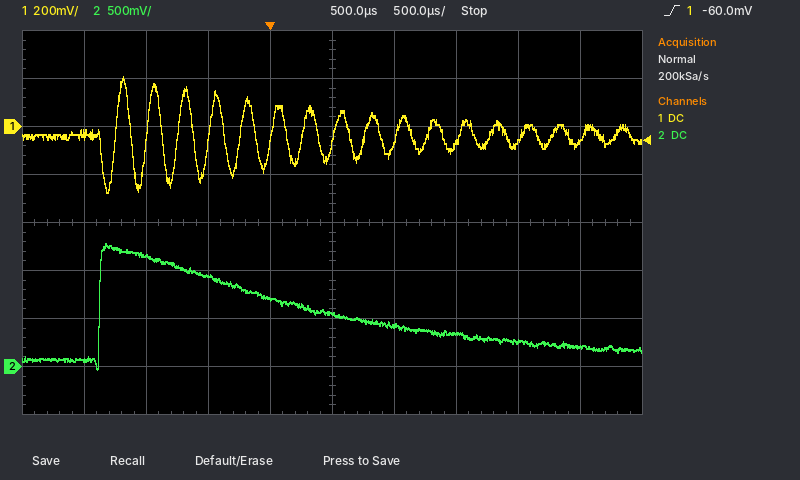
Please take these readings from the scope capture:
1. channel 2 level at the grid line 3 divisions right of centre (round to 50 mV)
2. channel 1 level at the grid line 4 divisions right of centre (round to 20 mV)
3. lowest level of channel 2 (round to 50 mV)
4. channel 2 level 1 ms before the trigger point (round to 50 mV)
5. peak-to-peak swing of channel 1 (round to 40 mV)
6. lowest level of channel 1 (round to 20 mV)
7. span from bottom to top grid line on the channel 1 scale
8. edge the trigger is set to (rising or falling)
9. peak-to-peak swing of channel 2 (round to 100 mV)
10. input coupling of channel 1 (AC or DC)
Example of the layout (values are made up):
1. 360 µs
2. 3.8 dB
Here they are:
1. 250 mV
2. -60 mV
3. -50 mV
4. 1.15 V
5. 480 mV
6. -280 mV
7. 1.6 V
8. rising
9. 1.30 V
10. DC
